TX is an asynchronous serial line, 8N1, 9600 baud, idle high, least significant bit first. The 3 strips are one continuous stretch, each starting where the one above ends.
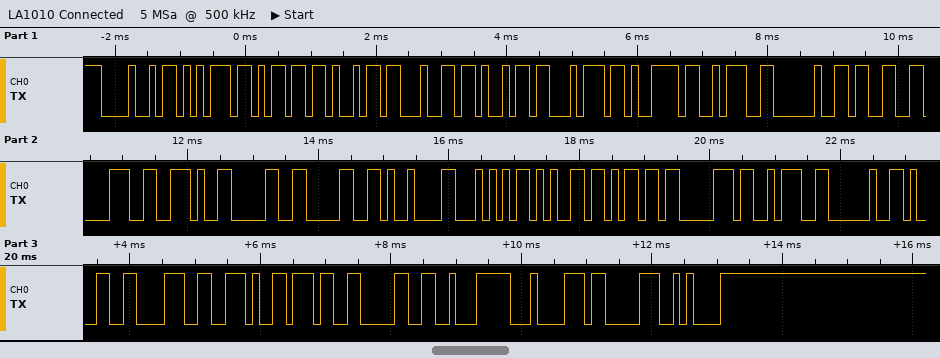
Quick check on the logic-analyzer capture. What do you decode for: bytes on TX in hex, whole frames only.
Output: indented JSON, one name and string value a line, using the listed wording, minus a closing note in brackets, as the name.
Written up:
{
  "bytes on TX in hex, whole frames only": "48 75 6D 69 64 69 74 79 3A 20 33 38 2E 30 30 09 54 65 6D 70 3A 20 31 38 2E 37 30 E2 84 83 0A"
}
